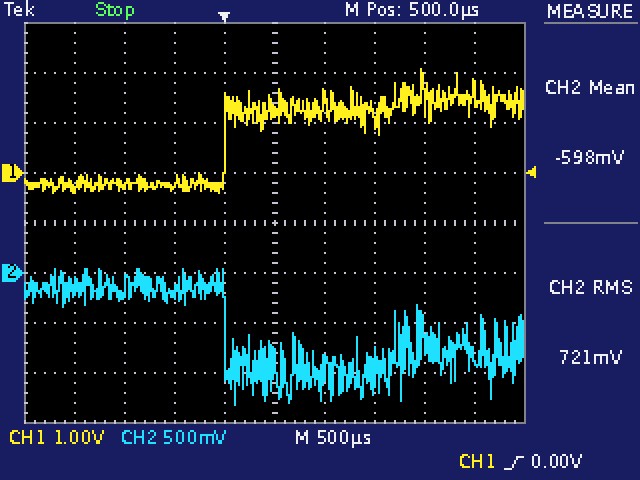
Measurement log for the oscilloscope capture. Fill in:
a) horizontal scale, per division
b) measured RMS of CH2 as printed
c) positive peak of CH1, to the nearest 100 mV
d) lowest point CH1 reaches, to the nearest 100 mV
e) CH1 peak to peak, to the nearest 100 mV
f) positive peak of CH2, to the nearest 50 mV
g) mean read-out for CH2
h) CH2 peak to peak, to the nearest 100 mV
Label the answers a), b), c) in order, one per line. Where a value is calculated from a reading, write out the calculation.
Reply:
a) 500 µs
b) 721 mV
c) 2.1 V
d) -400 mV
e) 2.1 V − (-400 mV) = 2.5 V
f) 50 mV
g) -598 mV
h) 1.40 V
